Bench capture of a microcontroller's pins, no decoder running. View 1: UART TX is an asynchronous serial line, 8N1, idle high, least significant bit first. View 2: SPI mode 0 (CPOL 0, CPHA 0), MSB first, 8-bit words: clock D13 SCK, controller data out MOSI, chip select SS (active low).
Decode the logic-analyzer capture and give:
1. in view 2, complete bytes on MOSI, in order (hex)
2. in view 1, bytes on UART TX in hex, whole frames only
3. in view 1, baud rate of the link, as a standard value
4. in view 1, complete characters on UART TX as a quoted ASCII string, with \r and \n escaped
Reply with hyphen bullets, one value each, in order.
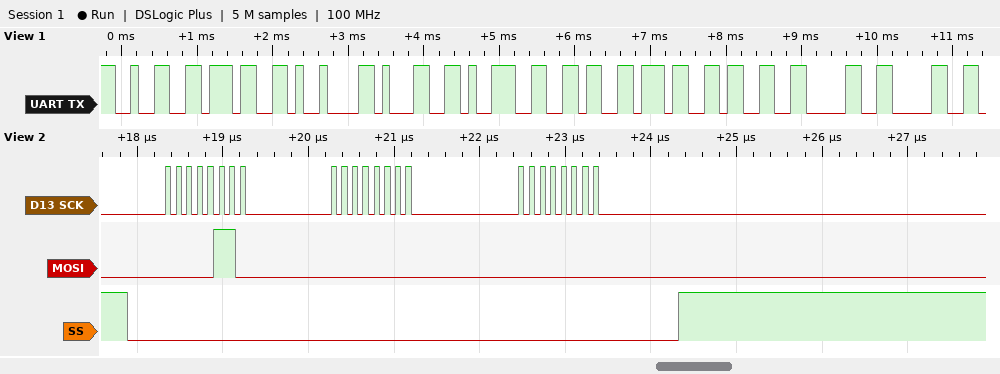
- 06 00 00
- 0x32 0x37 0x09 0x31 0x39 0x36 0x37 0x33 0x30 0x30
- 9600 baud
- "27\t1967300"
